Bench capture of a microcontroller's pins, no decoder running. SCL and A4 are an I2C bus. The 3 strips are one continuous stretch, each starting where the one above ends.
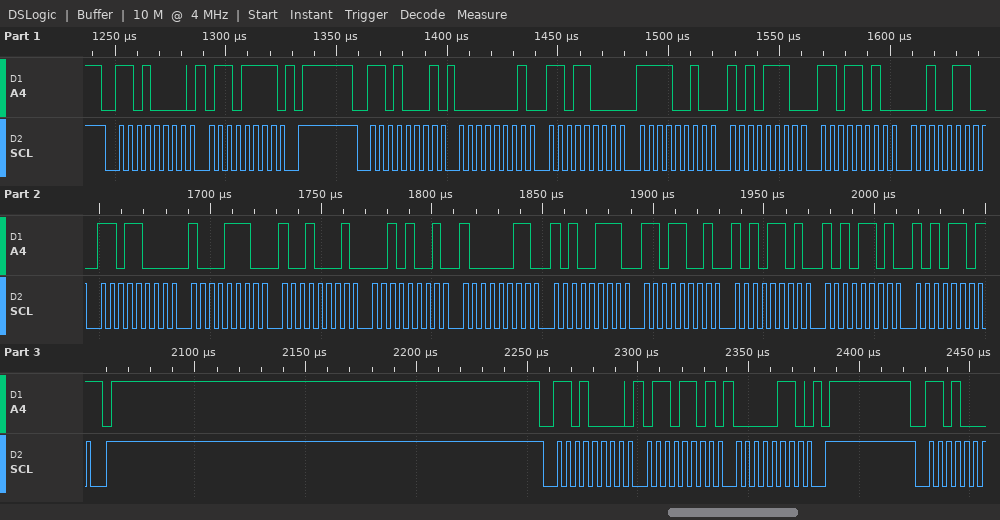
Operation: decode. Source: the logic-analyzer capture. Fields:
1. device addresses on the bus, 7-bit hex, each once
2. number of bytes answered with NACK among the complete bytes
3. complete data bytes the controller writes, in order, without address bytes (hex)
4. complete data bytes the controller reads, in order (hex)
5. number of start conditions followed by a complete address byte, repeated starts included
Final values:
0x68
1
6F 6D 06
01 D8 F2 AE DA 26 D8 8E 91 29 83 A7 D9 AD AD AD
3
